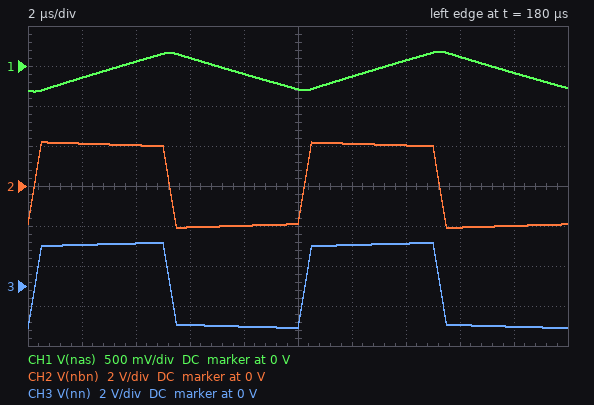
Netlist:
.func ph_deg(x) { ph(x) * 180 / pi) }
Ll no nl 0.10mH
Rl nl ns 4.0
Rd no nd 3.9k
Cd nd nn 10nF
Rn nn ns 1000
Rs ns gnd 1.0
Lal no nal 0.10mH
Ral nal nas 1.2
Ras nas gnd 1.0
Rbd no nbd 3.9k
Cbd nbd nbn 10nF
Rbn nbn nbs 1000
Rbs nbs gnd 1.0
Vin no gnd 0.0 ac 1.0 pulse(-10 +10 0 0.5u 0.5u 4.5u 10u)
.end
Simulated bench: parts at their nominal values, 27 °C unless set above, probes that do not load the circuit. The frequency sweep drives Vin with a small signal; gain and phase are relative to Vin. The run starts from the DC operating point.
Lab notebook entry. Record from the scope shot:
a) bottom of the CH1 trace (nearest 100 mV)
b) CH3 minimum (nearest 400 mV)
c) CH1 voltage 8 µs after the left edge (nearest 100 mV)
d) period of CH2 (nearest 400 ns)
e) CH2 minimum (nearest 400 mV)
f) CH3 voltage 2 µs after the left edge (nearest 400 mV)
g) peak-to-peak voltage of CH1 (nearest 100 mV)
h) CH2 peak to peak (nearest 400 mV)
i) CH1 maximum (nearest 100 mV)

-300 mV
-2.0 V
-100 mV
10.0 µs
-2.0 V
2.0 V
500 mV
4.4 V
200 mV
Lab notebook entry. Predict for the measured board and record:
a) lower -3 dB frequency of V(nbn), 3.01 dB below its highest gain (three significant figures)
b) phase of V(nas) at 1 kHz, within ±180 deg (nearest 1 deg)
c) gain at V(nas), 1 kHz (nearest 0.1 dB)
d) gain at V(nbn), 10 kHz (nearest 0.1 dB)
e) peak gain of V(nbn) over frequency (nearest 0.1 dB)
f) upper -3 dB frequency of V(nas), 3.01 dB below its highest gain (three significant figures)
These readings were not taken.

3.25 kHz
-16 deg
-7.2 dB
-14.2 dB
-13.8 dB
3.50 kHz
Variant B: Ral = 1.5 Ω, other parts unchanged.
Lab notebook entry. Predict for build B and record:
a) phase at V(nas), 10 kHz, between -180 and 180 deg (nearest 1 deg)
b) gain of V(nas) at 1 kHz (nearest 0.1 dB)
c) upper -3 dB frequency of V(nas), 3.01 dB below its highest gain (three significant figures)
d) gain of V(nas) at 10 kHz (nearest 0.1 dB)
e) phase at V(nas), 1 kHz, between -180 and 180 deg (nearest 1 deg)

-68 deg
-8.2 dB
3.98 kHz
-16.6 dB
-14 deg
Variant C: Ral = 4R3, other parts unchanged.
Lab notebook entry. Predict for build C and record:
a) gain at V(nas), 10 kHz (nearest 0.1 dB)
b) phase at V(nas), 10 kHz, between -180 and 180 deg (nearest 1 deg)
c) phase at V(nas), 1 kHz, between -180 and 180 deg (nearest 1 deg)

-18.3 dB
-50 deg
-7 deg
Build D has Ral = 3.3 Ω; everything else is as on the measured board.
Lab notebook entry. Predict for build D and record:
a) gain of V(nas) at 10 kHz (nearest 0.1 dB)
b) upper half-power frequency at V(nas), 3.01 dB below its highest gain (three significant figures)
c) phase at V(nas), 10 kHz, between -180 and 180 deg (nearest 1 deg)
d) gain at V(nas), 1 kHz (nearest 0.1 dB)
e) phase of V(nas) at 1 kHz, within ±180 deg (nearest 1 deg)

-17.6 dB
6.84 kHz
-56 deg
-12.8 dB
-8 deg
